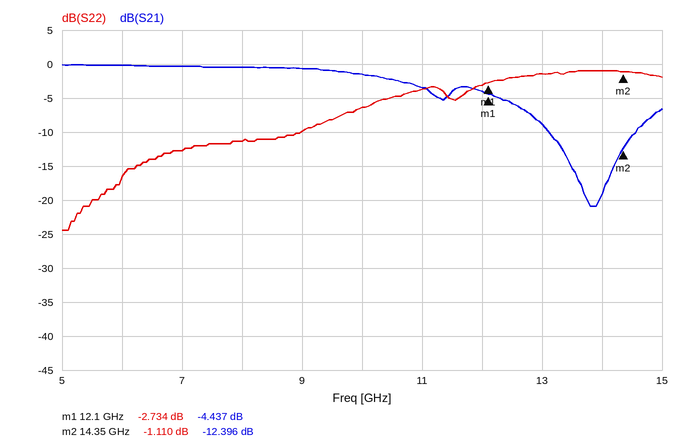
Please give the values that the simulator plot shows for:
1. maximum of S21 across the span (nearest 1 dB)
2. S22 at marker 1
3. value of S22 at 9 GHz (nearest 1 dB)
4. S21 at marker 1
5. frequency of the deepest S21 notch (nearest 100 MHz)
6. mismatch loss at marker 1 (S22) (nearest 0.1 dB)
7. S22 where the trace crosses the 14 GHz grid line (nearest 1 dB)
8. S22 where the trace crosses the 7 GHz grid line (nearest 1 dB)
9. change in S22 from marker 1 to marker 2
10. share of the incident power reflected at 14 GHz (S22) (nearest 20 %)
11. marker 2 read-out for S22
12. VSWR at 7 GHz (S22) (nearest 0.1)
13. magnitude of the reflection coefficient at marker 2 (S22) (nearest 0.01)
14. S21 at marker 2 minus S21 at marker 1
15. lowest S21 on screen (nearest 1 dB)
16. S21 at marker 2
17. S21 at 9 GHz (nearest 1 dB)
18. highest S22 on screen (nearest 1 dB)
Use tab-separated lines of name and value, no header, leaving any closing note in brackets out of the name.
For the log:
maximum of S21 across the span	0 dB
S22 at marker 1	-2.734 dB
value of S22 at 9 GHz	-10 dB
S21 at marker 1	-4.437 dB
frequency of the deepest S21 notch	13.8 GHz
mismatch loss at marker 1 (S22)	3.3 dB
S22 where the trace crosses the 14 GHz grid line	-1 dB
S22 where the trace crosses the 7 GHz grid line	-13 dB
change in S22 from marker 1 to marker 2	1.624 dB
share of the incident power reflected at 14 GHz (S22)	80 %
marker 2 read-out for S22	-1.110 dB
VSWR at 7 GHz (S22)	1.6
magnitude of the reflection coefficient at marker 2 (S22)	0.88
S21 at marker 2 minus S21 at marker 1	-7.959 dB
lowest S21 on screen	-21 dB
S21 at marker 2	-12.396 dB
S21 at 9 GHz	-1 dB
highest S22 on screen	-1 dB
